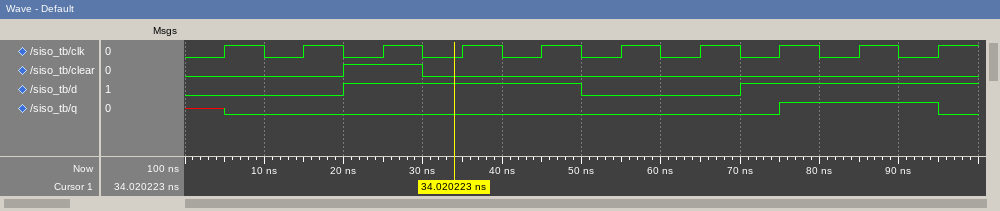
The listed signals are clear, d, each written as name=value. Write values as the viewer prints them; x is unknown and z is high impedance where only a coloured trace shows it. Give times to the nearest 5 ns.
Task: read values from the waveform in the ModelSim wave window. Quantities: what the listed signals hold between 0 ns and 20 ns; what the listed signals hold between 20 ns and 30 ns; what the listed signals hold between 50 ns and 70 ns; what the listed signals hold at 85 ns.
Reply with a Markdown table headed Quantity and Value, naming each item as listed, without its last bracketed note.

| Quantity | Value |
|---|---|
| what the listed signals hold between 0 ns and 20 ns | clear=0, d=0 |
| what the listed signals hold between 20 ns and 30 ns | clear=1, d=1 |
| what the listed signals hold between 50 ns and 70 ns | clear=0, d=0 |
| what the listed signals hold at 85 ns | clear=0, d=1 |
